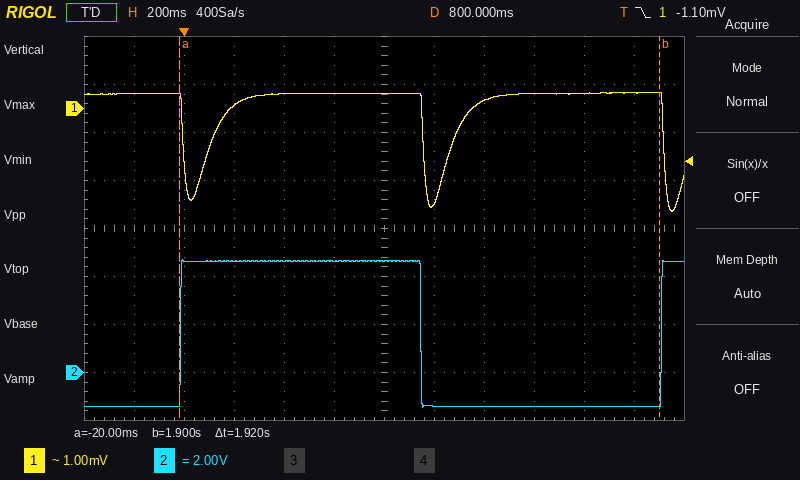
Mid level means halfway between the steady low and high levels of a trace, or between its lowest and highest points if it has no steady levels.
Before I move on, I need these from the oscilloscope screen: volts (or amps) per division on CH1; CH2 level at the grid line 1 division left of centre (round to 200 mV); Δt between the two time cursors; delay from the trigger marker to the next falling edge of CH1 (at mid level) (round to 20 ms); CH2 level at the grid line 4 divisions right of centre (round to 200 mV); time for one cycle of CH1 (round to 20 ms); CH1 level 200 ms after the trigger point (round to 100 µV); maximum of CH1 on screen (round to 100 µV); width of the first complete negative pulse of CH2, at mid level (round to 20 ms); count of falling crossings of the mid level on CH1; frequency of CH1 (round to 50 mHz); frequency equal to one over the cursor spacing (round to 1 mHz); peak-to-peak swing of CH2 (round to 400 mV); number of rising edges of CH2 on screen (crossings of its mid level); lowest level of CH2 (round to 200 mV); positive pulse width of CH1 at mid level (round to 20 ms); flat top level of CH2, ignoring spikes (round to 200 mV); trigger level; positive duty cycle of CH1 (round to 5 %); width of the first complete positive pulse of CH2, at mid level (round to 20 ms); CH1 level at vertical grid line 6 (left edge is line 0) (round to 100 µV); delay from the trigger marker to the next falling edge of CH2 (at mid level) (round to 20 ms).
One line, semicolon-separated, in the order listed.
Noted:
1 mV; 4.6 V; 1.92 s; 960 ms; -1.4 V; 960 ms; 100 µV; 300 µV; 960 ms; 3; 1.05 Hz; 521 mHz; 6.0 V; 2; -1.4 V; 860 ms; 4.6 V; -1.10 mV; 90 %; 960 ms; 300 µV; 940 ms
